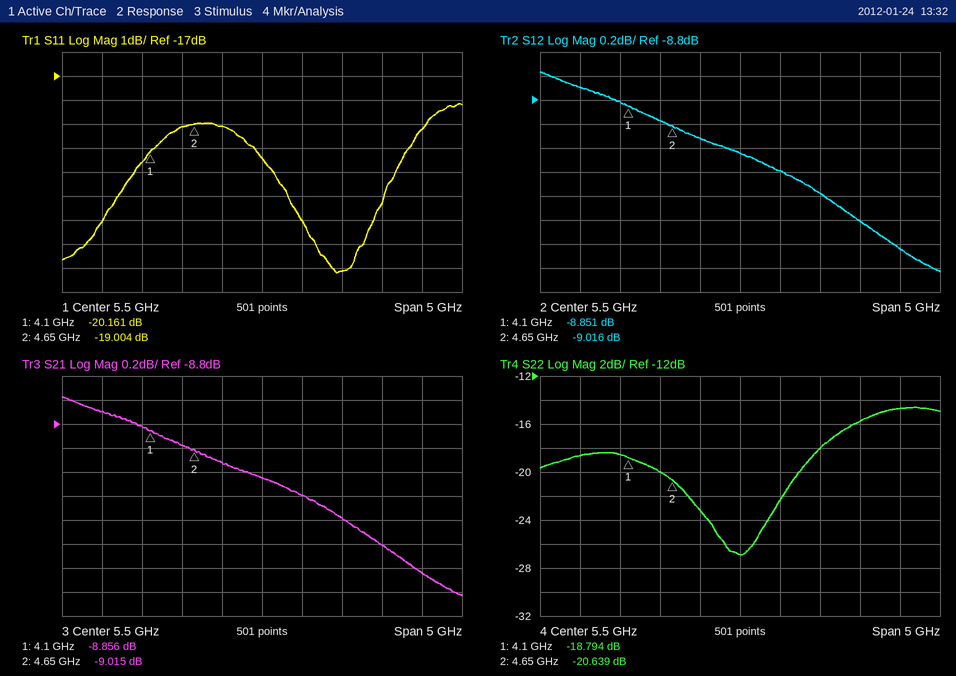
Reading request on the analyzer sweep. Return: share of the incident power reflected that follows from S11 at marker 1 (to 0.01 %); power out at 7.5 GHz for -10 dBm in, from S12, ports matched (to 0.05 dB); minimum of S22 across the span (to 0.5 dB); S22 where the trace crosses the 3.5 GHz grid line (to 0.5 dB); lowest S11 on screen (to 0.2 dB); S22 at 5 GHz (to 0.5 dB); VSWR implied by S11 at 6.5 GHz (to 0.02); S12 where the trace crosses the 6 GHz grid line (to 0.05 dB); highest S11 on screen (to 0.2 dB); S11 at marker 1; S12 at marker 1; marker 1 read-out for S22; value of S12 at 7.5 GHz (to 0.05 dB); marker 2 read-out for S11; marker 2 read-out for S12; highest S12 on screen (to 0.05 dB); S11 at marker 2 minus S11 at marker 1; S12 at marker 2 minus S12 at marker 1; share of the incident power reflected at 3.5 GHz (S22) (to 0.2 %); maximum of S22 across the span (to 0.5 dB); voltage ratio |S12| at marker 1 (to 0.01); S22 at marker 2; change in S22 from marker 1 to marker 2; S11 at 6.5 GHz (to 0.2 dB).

0.96 %
-20.05 dBm
-27.0 dB
-18.5 dB
-25.2 dB
-23.0 dB
1.12
-9.40 dB
-18.2 dB
-20.161 dB
-8.851 dB
-18.794 dB
-10.05 dB
-19.004 dB
-9.016 dB
-8.55 dB
1.157 dB
-0.165 dB
1.4 %
-14.5 dB
0.36
-20.639 dB
-1.845 dB
-25.2 dB
